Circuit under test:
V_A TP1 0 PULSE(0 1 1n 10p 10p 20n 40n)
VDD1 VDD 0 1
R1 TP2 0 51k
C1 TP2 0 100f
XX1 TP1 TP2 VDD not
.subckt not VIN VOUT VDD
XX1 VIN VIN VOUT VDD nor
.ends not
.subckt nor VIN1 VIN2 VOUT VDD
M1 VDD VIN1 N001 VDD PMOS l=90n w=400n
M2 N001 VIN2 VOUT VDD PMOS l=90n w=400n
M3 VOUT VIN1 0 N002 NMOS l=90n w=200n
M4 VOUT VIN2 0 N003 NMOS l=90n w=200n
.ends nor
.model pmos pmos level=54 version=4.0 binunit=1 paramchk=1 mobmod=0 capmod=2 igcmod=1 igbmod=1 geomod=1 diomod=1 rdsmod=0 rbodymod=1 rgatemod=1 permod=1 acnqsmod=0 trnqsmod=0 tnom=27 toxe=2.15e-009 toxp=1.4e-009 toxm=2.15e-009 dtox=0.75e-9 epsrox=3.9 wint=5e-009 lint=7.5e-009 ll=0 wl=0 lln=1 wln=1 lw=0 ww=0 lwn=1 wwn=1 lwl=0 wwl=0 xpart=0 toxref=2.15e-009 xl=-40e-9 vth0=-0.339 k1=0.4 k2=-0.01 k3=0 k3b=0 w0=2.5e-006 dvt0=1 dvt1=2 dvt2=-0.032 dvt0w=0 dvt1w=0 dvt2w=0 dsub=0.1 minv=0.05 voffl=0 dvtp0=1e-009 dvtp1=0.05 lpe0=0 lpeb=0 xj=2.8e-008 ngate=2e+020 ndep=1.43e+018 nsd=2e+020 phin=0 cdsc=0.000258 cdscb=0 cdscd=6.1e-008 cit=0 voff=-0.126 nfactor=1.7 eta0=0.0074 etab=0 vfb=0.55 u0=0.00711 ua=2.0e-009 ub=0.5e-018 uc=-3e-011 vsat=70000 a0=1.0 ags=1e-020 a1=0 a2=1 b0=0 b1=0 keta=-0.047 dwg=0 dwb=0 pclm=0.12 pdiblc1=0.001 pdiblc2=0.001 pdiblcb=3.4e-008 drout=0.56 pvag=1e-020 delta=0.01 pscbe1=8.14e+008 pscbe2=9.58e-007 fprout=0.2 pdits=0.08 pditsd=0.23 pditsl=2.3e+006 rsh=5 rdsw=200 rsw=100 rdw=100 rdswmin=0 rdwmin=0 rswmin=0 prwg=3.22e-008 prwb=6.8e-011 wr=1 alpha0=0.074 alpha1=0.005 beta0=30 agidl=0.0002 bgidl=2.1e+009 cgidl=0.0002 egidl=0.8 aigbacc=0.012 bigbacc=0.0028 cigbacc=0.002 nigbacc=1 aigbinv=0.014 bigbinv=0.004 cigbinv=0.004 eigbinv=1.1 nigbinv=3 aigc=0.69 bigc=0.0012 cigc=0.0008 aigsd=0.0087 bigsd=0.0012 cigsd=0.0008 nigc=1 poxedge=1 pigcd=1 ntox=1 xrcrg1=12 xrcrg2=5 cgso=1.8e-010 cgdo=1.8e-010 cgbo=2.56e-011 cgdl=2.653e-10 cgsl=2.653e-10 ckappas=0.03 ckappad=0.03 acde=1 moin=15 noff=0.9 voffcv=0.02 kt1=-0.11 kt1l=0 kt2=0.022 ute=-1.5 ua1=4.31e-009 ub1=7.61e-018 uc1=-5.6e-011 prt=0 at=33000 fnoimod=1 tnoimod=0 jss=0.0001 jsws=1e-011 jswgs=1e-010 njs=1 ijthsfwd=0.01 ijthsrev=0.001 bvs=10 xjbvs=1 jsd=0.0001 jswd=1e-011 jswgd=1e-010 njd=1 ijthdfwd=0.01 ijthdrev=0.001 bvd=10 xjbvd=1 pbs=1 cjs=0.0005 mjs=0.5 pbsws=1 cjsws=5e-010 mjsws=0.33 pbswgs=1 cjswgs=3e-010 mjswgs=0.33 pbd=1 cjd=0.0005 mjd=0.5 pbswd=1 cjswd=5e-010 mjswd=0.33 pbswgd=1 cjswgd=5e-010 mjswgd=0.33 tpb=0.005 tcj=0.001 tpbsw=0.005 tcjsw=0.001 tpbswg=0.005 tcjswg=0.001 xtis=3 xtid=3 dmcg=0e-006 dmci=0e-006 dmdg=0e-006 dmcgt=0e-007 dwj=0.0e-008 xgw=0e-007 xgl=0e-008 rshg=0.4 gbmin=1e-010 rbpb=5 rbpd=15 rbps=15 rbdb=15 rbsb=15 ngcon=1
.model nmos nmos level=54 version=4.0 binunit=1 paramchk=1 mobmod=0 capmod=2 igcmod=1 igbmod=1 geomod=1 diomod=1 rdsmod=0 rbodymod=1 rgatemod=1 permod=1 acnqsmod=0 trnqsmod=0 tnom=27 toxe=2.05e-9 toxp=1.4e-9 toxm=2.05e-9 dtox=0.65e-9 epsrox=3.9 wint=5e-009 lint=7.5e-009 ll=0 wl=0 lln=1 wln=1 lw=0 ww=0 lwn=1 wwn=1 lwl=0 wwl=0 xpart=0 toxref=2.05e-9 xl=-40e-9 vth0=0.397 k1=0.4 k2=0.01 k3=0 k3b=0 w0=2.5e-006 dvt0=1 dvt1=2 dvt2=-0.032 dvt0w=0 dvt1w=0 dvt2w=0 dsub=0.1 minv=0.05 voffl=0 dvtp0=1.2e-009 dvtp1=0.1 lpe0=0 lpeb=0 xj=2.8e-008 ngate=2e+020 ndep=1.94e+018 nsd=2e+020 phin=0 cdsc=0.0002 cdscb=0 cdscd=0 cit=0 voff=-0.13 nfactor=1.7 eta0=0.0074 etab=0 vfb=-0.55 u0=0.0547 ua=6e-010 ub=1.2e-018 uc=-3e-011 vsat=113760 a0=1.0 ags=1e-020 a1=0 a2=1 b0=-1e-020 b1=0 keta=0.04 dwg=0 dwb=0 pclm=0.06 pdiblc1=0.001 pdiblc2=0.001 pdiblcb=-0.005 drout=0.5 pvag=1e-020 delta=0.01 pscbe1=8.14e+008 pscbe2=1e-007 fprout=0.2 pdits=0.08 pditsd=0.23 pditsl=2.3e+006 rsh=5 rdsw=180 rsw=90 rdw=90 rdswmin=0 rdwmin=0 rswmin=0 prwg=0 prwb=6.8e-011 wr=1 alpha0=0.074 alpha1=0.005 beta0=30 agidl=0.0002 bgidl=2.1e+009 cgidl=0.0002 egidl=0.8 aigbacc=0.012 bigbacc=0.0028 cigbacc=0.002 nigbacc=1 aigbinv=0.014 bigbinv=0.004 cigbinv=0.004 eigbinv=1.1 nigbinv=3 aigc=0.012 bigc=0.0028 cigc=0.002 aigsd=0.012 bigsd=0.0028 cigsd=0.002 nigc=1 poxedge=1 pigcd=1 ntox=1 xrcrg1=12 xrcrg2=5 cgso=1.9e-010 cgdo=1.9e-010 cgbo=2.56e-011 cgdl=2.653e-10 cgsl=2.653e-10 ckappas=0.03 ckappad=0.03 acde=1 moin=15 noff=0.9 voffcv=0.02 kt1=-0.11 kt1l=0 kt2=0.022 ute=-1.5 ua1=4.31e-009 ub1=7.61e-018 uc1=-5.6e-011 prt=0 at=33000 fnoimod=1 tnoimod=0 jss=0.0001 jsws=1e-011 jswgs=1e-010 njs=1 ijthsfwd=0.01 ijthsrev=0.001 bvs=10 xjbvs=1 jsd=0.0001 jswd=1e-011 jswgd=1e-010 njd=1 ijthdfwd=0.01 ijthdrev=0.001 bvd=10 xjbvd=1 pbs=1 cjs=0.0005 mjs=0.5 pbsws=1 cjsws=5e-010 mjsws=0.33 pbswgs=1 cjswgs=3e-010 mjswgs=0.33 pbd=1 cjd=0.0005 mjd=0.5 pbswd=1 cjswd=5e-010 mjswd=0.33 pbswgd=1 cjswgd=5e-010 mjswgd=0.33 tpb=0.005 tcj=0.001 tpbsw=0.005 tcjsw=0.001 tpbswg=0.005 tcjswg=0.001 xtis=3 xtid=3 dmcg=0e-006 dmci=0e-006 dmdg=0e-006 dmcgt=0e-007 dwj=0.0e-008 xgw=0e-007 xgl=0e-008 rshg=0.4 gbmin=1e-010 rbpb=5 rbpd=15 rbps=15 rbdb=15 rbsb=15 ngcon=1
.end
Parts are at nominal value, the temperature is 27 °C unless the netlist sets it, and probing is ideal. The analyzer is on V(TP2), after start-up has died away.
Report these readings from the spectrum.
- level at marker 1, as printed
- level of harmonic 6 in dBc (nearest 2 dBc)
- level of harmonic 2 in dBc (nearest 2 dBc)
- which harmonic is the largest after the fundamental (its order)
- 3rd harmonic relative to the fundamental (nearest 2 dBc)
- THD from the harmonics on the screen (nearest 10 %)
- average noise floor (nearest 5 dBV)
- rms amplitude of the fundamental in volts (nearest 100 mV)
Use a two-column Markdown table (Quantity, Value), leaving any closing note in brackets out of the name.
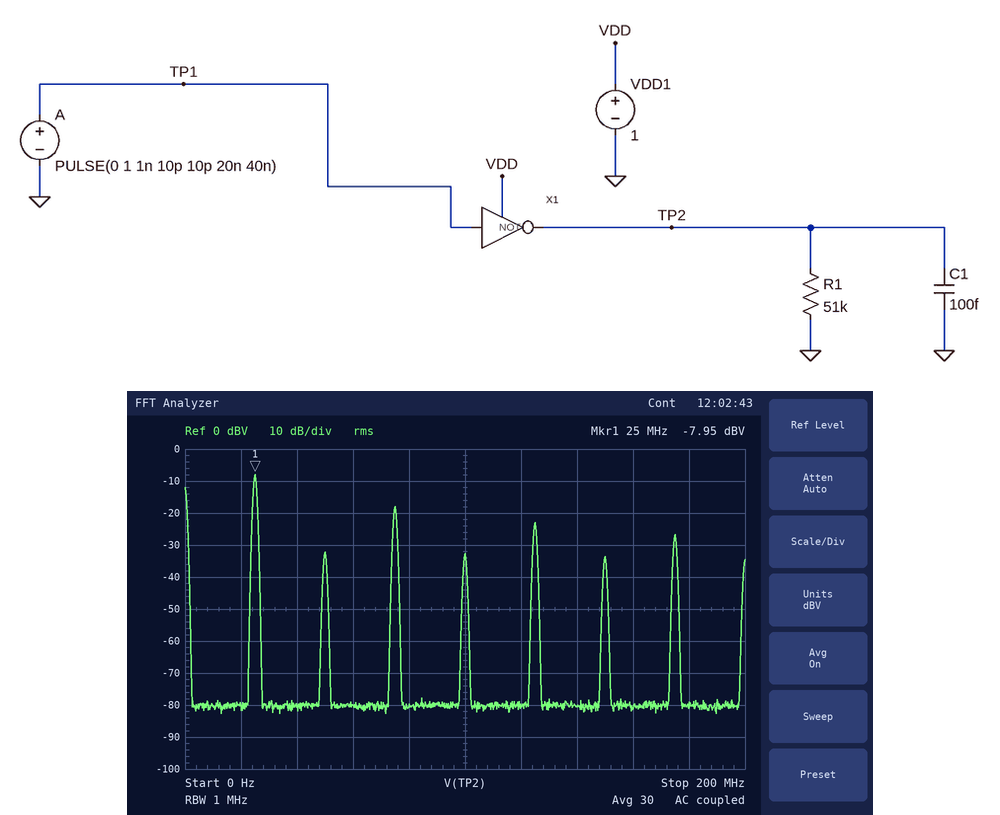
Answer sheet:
| Quantity | Value |
|---|---|
| level at marker 1, as printed | -7.95 dBV |
| level of harmonic 6 in dBc | -26 dBc |
| level of harmonic 2 in dBc | -24 dBc |
| which harmonic is the largest after the fundamental | 3 |
| 3rd harmonic relative to the fundamental | -10 dBc |
| THD from the harmonics on the screen | 40 % |
| average noise floor | -80 dBV |
| rms amplitude of the fundamental in volts | 400 mV |
